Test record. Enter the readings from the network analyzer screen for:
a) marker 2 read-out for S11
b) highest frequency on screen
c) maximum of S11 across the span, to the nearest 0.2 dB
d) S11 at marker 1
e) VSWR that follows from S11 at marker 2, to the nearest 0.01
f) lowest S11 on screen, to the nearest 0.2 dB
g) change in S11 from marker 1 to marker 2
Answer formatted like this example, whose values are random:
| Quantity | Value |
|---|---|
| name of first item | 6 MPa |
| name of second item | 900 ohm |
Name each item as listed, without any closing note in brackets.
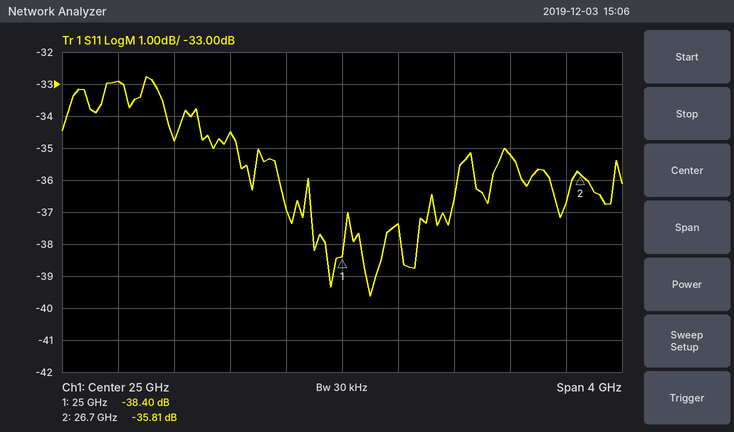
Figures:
| Quantity | Value |
|---|---|
| marker 2 read-out for S11 | -35.81 dB |
| highest frequency on screen | 27 GHz |
| maximum of S11 across the span, to the nearest 0.2 dB | -32.8 dB |
| S11 at marker 1 | -38.40 dB |
| VSWR that follows from S11 at marker 2, to the nearest 0.01 | 1.03 |
| lowest S11 on screen, to the nearest 0.2 dB | -39.6 dB |
| change in S11 from marker 1 to marker 2 | 2.59 dB |
